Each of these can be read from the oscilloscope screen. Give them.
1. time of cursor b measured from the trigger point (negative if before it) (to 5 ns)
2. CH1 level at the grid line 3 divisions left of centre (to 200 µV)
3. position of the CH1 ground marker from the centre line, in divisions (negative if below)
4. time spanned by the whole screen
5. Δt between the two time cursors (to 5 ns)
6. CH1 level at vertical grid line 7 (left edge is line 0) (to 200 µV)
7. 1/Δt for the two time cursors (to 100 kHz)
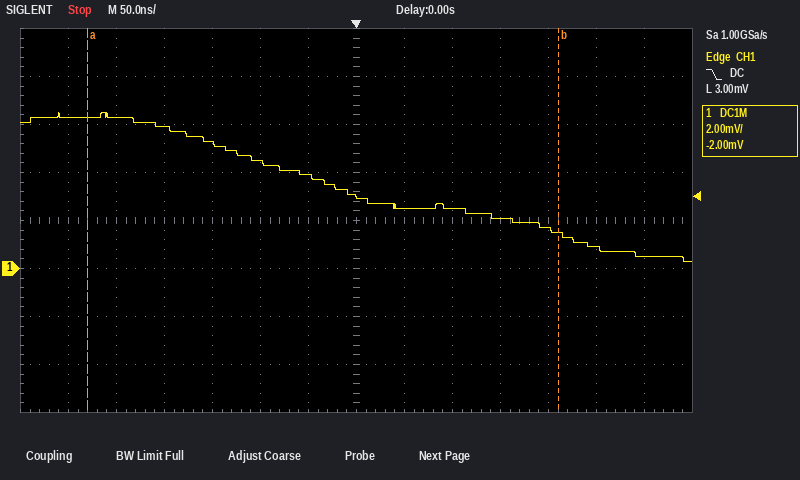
+210 ns
5.2 mV
-1.0 div
700 ns
490 ns
3.0 mV
2.0 MHz
